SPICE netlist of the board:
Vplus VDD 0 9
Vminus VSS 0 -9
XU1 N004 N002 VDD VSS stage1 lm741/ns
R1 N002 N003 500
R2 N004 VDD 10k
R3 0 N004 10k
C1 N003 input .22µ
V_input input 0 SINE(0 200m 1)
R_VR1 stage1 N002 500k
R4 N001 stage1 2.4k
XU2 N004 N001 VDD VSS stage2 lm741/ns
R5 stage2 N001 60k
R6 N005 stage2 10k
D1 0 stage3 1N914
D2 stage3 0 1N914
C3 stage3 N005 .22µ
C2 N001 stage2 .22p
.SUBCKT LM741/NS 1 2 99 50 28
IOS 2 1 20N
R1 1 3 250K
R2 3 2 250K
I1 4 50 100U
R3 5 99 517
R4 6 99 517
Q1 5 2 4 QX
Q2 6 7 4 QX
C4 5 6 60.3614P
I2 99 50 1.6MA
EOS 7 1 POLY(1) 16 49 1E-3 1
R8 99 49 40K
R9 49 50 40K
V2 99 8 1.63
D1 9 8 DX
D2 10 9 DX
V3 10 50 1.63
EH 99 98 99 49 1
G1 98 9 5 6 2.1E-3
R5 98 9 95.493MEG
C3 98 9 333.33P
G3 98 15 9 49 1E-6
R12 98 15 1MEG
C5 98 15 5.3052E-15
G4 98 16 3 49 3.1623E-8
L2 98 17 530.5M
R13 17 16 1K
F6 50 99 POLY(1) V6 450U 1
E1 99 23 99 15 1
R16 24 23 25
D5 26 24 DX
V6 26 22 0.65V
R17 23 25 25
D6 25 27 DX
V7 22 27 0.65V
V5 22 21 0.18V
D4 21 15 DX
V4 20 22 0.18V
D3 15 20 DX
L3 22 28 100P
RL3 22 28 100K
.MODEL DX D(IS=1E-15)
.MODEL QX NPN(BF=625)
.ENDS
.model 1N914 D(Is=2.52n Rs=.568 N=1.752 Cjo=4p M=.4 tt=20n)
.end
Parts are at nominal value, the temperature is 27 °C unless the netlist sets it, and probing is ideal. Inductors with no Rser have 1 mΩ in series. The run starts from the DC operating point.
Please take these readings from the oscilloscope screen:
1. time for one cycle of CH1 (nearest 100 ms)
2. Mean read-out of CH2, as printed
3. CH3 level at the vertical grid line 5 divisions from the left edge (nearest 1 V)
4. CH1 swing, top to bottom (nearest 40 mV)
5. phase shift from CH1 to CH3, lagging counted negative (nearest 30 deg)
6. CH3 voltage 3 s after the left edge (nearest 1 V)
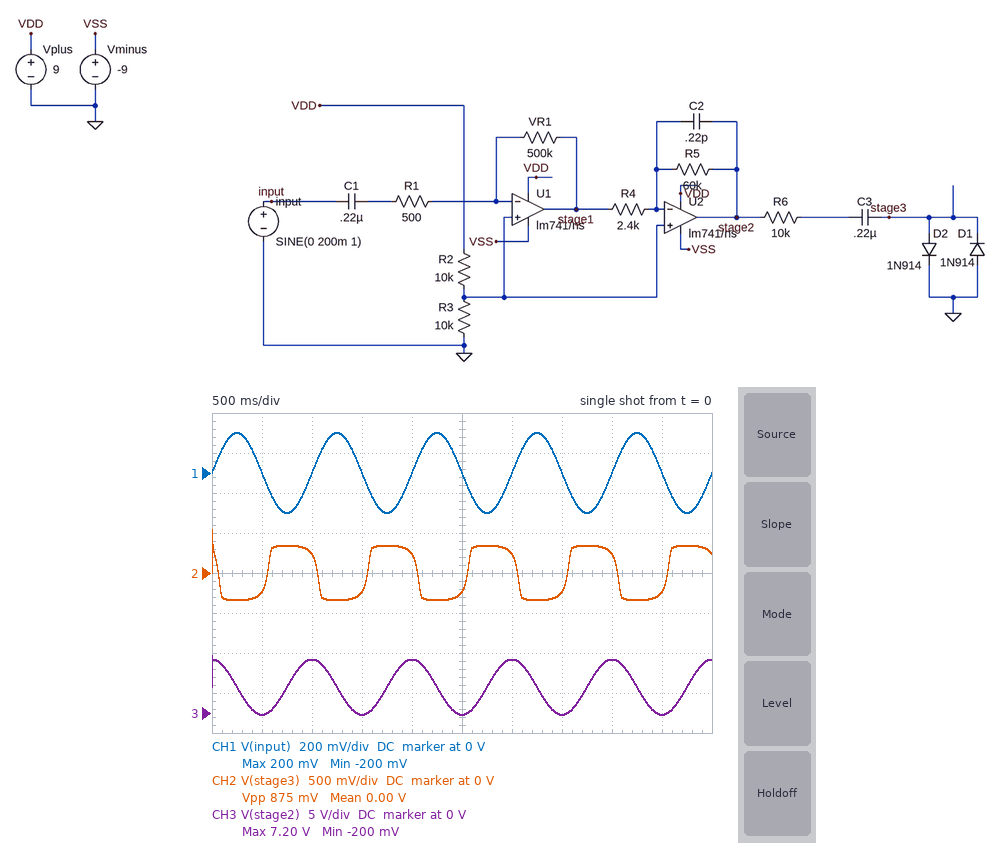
1.0 s
0.00 V
0 V
400 mV
90 deg
7 V
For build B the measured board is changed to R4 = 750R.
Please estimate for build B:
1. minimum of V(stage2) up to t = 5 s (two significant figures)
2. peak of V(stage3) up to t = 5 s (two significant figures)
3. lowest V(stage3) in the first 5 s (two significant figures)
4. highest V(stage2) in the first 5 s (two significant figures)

-8.0 V
600 mV
-590 mV
8.0 V
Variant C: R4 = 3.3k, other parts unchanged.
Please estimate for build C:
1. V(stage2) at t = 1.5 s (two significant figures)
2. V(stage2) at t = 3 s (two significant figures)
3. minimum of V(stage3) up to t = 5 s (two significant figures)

1.1 V
6.1 V
-330 mV
